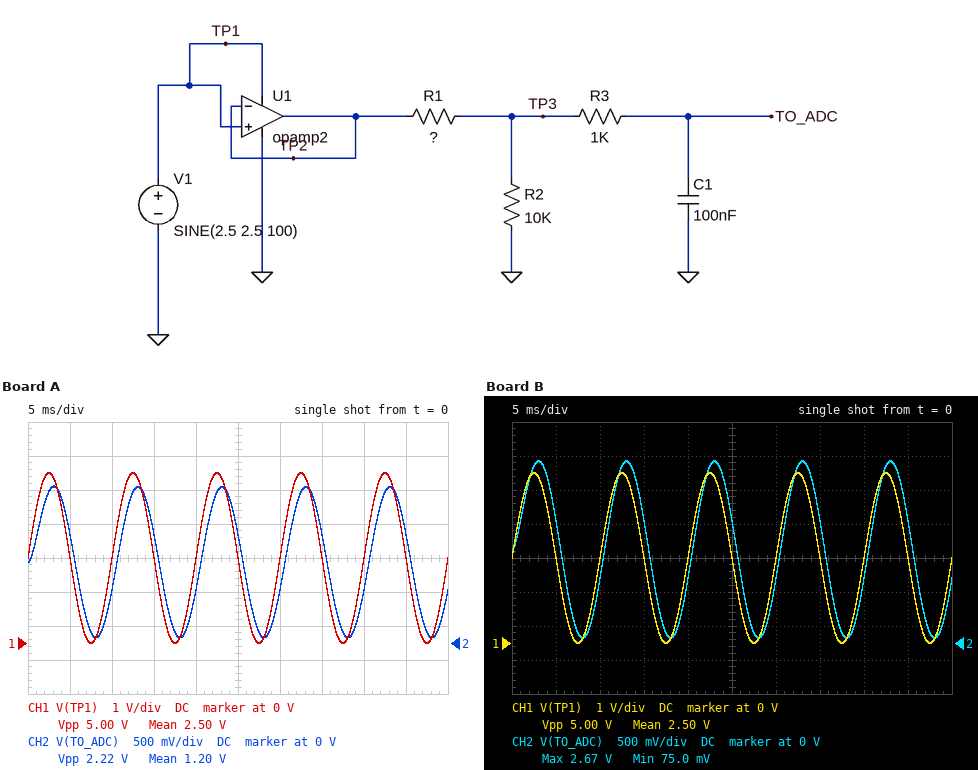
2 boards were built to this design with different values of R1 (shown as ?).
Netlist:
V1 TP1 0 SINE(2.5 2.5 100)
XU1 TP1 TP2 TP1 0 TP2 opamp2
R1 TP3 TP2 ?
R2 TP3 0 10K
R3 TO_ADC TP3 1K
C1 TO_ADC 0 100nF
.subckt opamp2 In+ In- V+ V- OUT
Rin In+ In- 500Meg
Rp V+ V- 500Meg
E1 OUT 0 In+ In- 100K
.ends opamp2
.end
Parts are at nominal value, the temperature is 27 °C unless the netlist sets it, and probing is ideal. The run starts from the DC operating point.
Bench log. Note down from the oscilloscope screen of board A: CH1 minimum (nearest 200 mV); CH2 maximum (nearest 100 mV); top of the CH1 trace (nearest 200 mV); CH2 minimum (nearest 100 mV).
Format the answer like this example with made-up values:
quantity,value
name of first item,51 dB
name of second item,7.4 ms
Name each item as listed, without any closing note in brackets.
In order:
quantity,value
CH1 minimum,0 V
CH2 maximum,2.3 V
top of the CH1 trace,5.0 V
CH2 minimum,100 mV
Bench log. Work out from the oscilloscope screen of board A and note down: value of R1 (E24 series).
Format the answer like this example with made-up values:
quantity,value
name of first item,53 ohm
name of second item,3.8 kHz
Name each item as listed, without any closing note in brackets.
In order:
quantity,value
value of R1,11 kΩ
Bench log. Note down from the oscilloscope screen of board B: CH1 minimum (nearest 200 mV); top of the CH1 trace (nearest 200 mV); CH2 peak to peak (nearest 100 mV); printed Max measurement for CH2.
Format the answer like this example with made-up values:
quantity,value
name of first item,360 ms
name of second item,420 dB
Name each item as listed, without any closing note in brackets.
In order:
quantity,value
CH1 minimum,0 V
top of the CH1 trace,5.0 V
CH2 peak to peak,2.6 V
printed Max measurement for CH2,2.67 V
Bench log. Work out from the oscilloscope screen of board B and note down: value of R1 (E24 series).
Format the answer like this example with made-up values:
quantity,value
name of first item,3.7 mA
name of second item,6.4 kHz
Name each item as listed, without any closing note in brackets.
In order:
quantity,value
value of R1,8.2 kΩ
